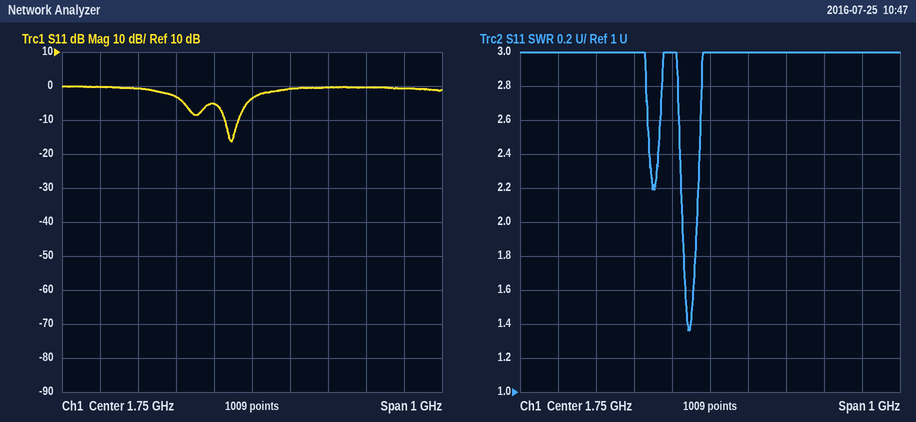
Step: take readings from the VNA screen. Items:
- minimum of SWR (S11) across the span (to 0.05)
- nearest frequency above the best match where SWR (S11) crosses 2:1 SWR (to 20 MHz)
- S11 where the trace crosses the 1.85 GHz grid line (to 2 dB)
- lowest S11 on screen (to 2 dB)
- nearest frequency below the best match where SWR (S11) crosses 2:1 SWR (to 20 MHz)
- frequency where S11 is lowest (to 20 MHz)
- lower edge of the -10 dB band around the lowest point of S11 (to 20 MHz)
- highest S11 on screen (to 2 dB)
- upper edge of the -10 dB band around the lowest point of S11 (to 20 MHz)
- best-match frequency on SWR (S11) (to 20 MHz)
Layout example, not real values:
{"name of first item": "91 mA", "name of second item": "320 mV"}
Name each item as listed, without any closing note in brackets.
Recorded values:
{"minimum of SWR (S11) across the span": "1.35", "nearest frequency above the best match where SWR (S11) crosses 2:1 SWR": "1.72 GHz", "S11 where the trace crosses the 1.85 GHz grid line": "0 dB", "lowest S11 on screen": "-16 dB", "nearest frequency below the best match where SWR (S11) crosses 2:1 SWR": "1.68 GHz", "frequency where S11 is lowest": "1.70 GHz", "lower edge of the -10 dB band around the lowest point of S11": "1.68 GHz", "highest S11 on screen": "0 dB", "upper edge of the -10 dB band around the lowest point of S11": "1.72 GHz", "best-match frequency on SWR (S11)": "1.70 GHz"}
